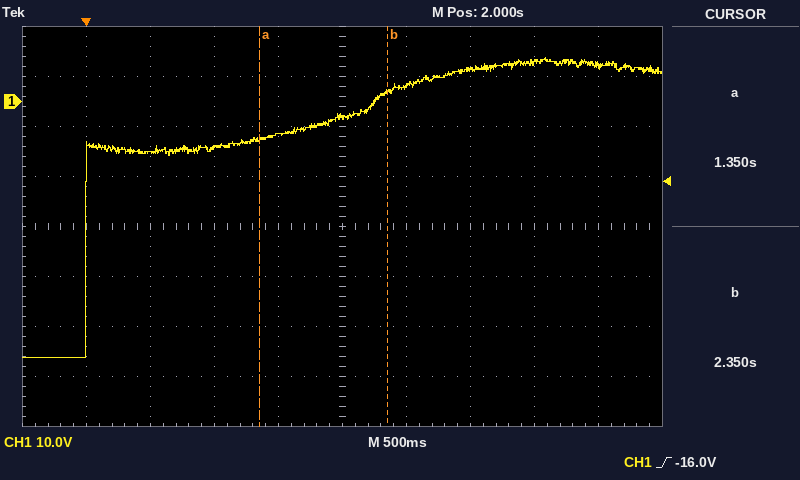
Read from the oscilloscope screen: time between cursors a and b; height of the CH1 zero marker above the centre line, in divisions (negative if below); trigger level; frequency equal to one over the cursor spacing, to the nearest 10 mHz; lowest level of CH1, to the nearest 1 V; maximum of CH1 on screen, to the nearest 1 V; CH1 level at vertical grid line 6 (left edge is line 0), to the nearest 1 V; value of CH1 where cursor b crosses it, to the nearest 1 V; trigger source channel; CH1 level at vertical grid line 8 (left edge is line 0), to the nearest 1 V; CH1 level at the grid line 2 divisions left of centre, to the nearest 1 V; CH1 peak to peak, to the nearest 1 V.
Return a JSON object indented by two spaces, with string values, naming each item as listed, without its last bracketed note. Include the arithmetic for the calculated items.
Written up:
{
  "time between cursors a and b": "2.35 s − (1.35 s) = 1.00 s",
  "height of the CH1 zero marker above the centre line, in divisions": "+2.5 div",
  "trigger level": "-16.0 V",
  "frequency equal to one over the cursor spacing, to the nearest 10 mHz": "1 / 1.00 s ≈ 1.00 Hz",
  "lowest level of CH1, to the nearest 1 V": "-51 V",
  "maximum of CH1 on screen, to the nearest 1 V": "9 V",
  "CH1 level at vertical grid line 6 (left edge is line 0), to the nearest 1 V": "3 V",
  "value of CH1 where cursor b crosses it, to the nearest 1 V": "2 V",
  "trigger source channel": "CH1",
  "CH1 level at vertical grid line 8 (left edge is line 0), to the nearest 1 V": "8 V",
  "CH1 level at the grid line 2 divisions left of centre, to the nearest 1 V": "-9 V",
  "CH1 peak to peak, to the nearest 1 V": "9 V − (-51 V) = 60 V"
}
